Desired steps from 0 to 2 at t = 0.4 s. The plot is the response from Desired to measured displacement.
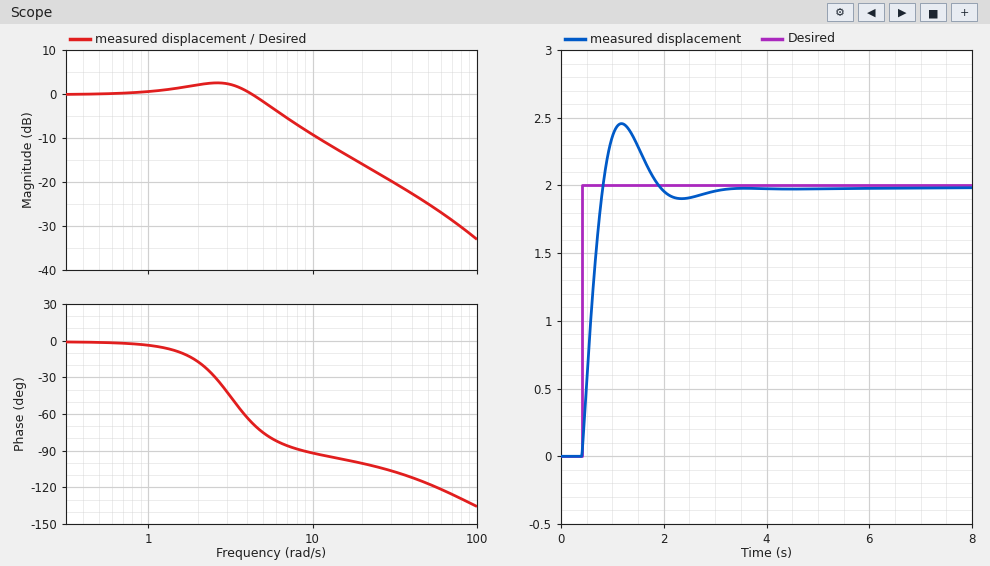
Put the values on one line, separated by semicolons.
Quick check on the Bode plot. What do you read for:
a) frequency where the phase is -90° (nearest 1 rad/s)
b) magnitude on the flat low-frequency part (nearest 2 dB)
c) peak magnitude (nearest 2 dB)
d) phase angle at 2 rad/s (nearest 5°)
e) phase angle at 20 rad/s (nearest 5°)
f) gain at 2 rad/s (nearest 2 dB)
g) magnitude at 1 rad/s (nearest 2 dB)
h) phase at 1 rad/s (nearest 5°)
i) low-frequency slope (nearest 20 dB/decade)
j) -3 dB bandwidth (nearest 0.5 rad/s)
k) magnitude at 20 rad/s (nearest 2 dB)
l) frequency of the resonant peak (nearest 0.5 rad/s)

9 rad/s; 0 dB; 2 dB; -15°; -100°; 2 dB; 0 dB; -5°; 0 dB/decade; 5.5 rad/s; -16 dB; 2.5 rad/s
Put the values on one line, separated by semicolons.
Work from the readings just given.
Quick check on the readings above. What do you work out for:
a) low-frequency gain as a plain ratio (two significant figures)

1.0
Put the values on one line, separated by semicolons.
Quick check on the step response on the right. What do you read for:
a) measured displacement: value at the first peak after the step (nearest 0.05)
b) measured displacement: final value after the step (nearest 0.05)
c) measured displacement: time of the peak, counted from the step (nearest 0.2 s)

2.45; 2.00; 0.8 s
